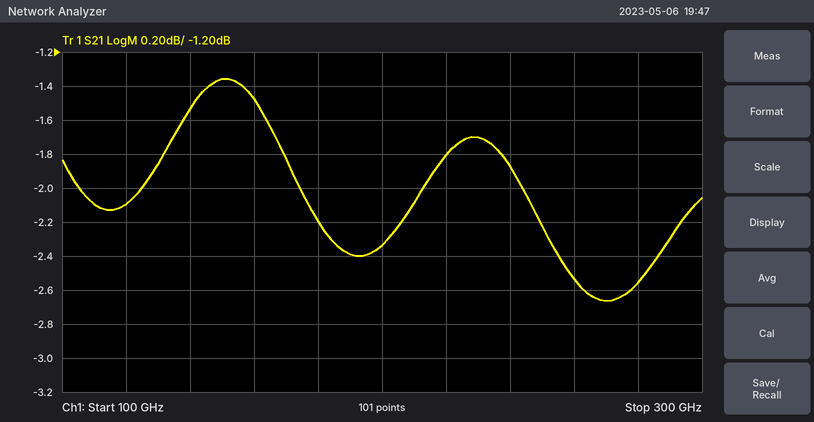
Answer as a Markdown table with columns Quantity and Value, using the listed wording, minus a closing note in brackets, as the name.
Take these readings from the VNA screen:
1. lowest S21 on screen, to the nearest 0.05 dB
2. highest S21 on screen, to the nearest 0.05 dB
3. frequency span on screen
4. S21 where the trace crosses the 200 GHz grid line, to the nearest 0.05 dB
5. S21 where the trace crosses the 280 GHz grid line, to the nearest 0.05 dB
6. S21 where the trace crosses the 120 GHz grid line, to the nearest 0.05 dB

| Quantity | Value |
|---|---|
| lowest S21 on screen, to the nearest 0.05 dB | -2.65 dB |
| highest S21 on screen, to the nearest 0.05 dB | -1.35 dB |
| frequency span on screen | 200 GHz |
| S21 where the trace crosses the 200 GHz grid line, to the nearest 0.05 dB | -2.35 dB |
| S21 where the trace crosses the 280 GHz grid line, to the nearest 0.05 dB | -2.55 dB |
| S21 where the trace crosses the 120 GHz grid line, to the nearest 0.05 dB | -2.10 dB |
